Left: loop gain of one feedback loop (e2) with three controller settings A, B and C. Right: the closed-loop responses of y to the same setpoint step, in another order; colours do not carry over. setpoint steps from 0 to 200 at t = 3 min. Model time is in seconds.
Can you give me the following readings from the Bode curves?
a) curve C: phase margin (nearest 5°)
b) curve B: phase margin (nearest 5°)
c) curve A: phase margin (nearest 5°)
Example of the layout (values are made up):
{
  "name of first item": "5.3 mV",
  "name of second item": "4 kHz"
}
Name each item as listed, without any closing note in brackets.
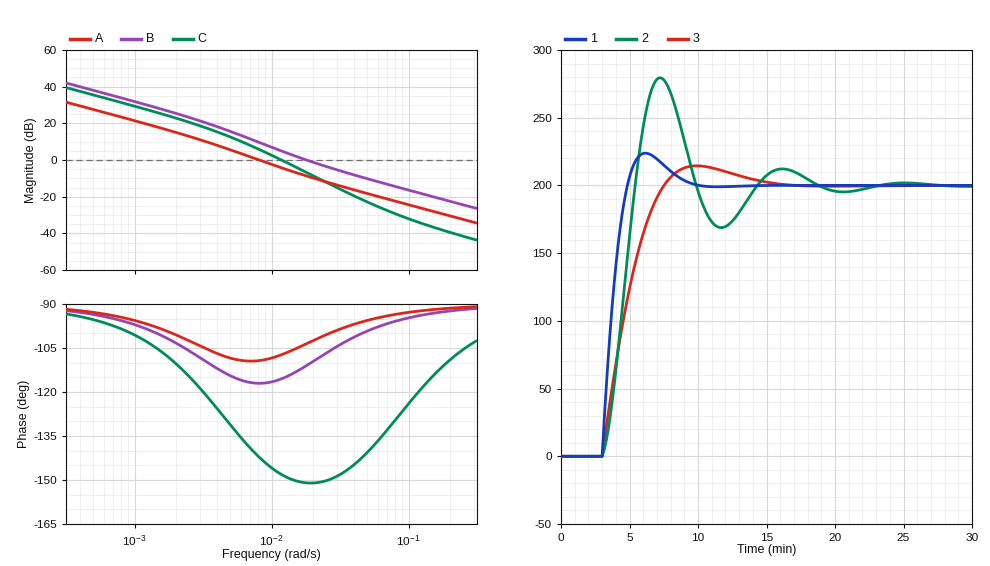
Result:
{
  "curve C: phase margin": "30°",
  "curve B: phase margin": "70°",
  "curve A: phase margin": "70°"
}
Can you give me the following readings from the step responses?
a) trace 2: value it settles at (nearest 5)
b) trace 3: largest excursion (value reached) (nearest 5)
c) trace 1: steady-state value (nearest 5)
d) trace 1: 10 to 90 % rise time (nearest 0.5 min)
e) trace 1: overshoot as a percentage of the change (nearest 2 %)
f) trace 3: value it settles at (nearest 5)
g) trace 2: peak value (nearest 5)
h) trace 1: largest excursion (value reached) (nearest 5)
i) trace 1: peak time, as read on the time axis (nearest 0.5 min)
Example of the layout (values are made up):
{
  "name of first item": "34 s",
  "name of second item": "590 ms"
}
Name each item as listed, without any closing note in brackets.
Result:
{
  "trace 2: value it settles at": "200",
  "trace 3: largest excursion (value reached)": "215",
  "trace 1: steady-state value": "200",
  "trace 1: 10 to 90 % rise time": "1.5 min",
  "trace 1: overshoot as a percentage of the change": "12 %",
  "trace 3: value it settles at": "200",
  "trace 2: peak value": "280",
  "trace 1: largest excursion (value reached)": "225",
  "trace 1: peak time, as read on the time axis": "6.0 min"
}
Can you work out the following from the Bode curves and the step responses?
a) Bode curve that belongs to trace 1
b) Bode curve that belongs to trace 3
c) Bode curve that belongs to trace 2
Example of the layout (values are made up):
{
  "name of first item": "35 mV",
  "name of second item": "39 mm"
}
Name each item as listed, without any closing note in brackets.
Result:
{
  "Bode curve that belongs to trace 1": "B",
  "Bode curve that belongs to trace 3": "A",
  "Bode curve that belongs to trace 2": "C"
}
